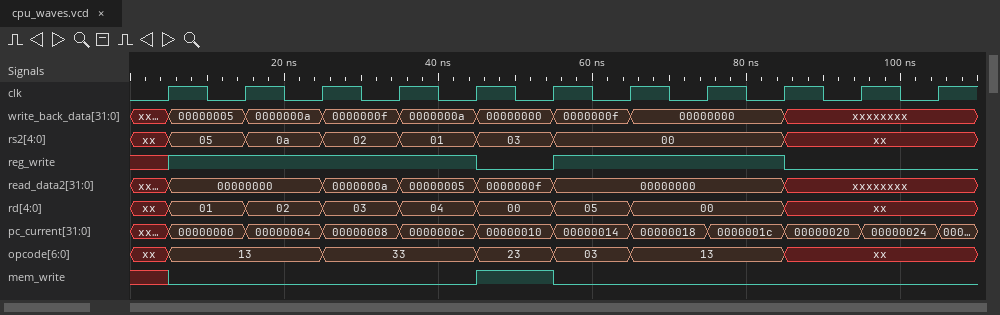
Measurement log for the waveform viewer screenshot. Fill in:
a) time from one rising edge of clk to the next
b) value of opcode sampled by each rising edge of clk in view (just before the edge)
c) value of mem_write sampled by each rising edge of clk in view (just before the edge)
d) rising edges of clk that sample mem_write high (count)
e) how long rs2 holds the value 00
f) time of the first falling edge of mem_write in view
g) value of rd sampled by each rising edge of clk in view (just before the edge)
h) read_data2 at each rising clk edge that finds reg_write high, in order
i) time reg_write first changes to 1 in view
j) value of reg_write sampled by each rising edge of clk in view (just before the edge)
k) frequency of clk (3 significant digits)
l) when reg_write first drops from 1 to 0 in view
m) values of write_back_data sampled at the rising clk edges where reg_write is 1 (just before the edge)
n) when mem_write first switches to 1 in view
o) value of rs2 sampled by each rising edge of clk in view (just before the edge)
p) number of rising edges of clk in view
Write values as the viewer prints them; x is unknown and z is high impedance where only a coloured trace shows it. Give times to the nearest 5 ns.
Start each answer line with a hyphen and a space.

- 10 ns
- xx, 13, 13, 33, 33, 23, 03, 13, 13, xx, xx
- x 0 0 0 0 1 0 0 0 0 0
- 1
- 30 ns
- 55 ns
- xx, 01, 02, 03, 04, 00, 05, 00, 00, xx, xx
- 00000000, 00000000, 0000000a, 00000005, 00000000, 00000000, 00000000
- 5 ns
- x 1 1 1 1 0 1 1 1 0 0
- 100 MHz
- 45 ns
- 00000005, 0000000a, 0000000f, 0000000a, 0000000f, 00000000, 00000000
- 45 ns
- xx, 05, 0a, 02, 01, 03, 00, 00, 00, xx, xx
- 11
